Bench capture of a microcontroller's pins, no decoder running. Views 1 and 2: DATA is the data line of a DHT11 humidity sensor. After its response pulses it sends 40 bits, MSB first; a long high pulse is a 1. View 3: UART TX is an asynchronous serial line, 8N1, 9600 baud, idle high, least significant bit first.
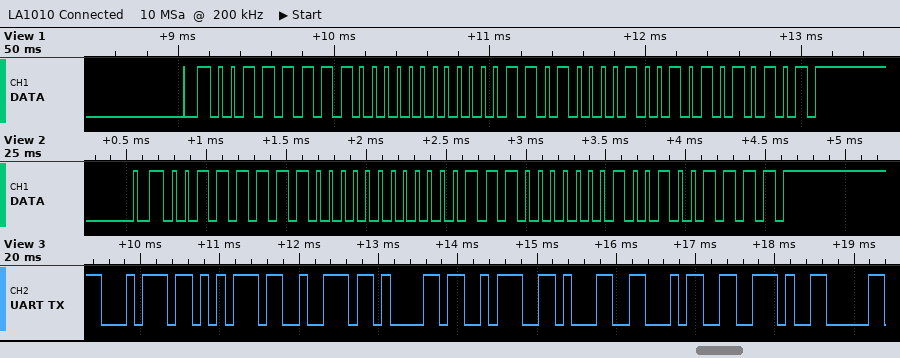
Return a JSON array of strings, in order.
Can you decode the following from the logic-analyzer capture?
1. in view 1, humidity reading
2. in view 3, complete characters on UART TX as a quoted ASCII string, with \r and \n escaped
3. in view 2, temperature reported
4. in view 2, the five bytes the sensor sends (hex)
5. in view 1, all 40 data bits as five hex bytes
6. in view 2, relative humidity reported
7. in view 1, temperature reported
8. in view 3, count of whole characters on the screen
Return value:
["63 %", "\"tura:14.\"", "14.2 °C", "3F 00 0E 02 4F", "3F 00 0D 09 55", "63 %", "13.9 °C", "8"]
